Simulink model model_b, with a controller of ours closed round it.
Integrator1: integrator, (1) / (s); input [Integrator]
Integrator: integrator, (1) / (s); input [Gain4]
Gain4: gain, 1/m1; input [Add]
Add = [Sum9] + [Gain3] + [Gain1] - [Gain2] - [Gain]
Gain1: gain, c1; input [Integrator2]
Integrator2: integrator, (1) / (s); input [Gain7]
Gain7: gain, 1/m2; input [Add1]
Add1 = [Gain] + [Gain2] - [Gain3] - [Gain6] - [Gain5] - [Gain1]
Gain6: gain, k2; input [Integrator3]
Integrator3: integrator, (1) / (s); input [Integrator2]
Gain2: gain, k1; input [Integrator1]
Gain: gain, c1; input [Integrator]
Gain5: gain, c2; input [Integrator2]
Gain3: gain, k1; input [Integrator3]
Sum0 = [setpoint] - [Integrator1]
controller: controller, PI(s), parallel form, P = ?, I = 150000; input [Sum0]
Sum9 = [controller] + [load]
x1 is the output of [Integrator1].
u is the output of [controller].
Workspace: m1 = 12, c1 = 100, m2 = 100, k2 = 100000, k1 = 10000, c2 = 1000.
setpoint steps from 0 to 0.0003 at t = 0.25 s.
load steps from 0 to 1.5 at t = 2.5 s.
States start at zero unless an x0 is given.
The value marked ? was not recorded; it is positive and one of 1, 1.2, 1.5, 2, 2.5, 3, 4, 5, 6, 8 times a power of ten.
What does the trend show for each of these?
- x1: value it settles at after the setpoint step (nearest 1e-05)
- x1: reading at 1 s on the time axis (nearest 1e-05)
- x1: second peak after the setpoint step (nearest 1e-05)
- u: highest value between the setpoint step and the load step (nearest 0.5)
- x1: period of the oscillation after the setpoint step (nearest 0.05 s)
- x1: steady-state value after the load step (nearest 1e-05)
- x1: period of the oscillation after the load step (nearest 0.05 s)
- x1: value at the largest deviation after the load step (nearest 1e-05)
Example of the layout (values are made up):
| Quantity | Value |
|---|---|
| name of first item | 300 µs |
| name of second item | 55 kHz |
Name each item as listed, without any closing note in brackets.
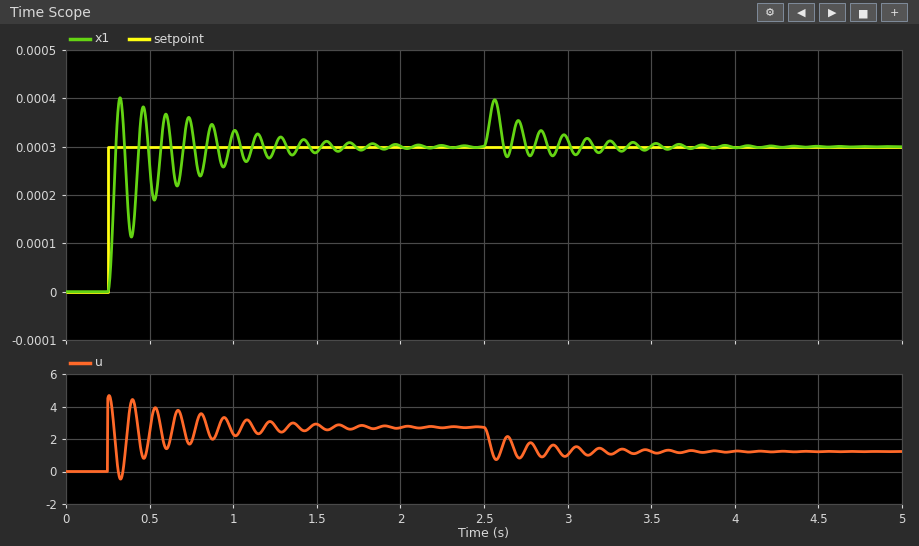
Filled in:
| Quantity | Value |
|---|---|
| x1: value it settles at after the setpoint step | 0.00030 |
| x1: reading at 1 s on the time axis | 0.00033 |
| x1: second peak after the setpoint step | 0.00038 |
| u: highest value between the setpoint step and the load step | 4.5 |
| x1: period of the oscillation after the setpoint step | 0.15 s |
| x1: steady-state value after the load step | 0.00030 |
| x1: period of the oscillation after the load step | 0.15 s |
| x1: value at the largest deviation after the load step | 0.00040 |
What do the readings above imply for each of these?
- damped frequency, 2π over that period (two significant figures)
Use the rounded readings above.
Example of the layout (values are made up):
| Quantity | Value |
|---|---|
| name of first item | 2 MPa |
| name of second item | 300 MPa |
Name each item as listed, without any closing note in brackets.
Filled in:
| Quantity | Value |
|---|---|
| damped frequency, 2π over that period | 42 rad/s |
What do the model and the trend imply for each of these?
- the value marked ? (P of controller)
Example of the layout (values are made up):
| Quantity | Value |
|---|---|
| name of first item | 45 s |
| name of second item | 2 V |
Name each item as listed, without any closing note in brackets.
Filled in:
| Quantity | Value |
|---|---|
| the value marked ? | 15000 |
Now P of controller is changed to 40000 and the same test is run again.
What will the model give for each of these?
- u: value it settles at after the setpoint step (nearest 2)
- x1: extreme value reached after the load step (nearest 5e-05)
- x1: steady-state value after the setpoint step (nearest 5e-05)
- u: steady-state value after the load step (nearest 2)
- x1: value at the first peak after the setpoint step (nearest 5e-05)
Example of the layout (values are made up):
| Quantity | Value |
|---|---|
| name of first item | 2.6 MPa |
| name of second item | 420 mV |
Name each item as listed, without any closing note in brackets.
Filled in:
| Quantity | Value |
|---|---|
| u: value it settles at after the setpoint step | 2 |
| x1: extreme value reached after the load step | 0.00035 |
| x1: steady-state value after the setpoint step | 0.00030 |
| u: steady-state value after the load step | 2 |
| x1: value at the first peak after the setpoint step | 0.00045 |
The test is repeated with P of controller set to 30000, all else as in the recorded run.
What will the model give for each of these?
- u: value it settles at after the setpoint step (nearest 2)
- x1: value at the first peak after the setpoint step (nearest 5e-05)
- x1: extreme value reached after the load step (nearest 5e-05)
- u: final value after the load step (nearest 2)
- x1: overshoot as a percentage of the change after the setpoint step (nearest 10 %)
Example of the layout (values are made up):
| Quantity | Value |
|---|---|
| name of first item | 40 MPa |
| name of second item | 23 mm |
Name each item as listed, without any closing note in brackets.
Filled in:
| Quantity | Value |
|---|---|
| u: value it settles at after the setpoint step | 2 |
| x1: value at the first peak after the setpoint step | 0.00045 |
| x1: extreme value reached after the load step | 0.00035 |
| u: final value after the load step | 2 |
| x1: overshoot as a percentage of the change after the setpoint step | 50 % |
